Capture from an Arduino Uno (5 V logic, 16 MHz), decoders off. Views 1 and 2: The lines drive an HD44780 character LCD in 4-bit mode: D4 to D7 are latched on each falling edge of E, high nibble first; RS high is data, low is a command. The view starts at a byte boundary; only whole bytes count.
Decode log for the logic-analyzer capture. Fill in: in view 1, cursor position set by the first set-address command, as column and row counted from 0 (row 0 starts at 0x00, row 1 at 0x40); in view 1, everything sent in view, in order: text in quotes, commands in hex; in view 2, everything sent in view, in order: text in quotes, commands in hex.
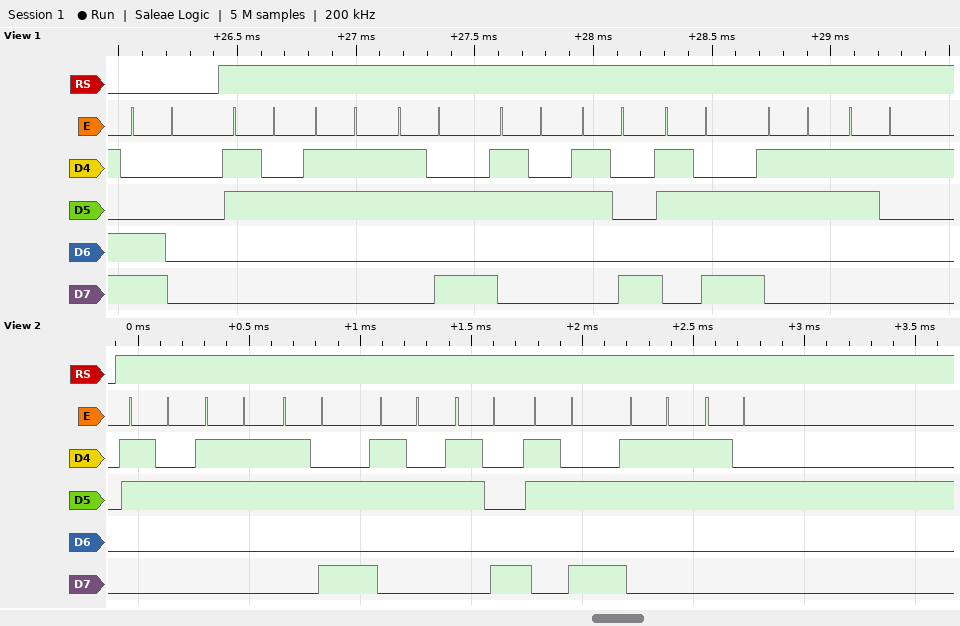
column 0, row 1
0xC0 "23:28:31"
"23:28:32"
